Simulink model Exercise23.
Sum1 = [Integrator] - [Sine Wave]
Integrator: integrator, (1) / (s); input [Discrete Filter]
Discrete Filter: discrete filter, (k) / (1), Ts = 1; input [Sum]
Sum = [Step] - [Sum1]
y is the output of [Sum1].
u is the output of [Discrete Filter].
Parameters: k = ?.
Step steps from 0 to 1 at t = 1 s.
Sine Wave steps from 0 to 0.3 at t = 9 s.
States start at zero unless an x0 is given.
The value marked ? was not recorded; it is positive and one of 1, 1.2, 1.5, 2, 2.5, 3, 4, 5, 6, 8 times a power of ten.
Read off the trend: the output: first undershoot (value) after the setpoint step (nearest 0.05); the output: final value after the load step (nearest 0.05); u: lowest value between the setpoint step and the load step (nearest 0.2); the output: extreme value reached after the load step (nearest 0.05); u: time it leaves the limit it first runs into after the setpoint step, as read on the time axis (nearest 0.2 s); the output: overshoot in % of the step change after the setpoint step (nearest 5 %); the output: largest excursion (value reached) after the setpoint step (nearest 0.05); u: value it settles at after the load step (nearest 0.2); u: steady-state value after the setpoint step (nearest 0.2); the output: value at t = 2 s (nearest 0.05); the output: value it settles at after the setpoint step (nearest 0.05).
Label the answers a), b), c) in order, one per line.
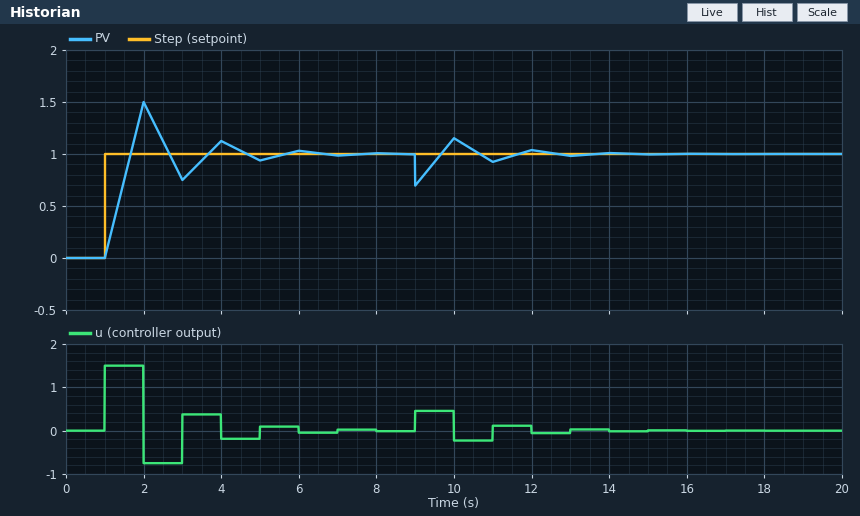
a) 0.75
b) 1.00
c) -0.8
d) 0.70
e) 2.0 s
f) 50 %
g) 1.50
h) 0.0
i) 0.0
j) 1.50
k) 1.00
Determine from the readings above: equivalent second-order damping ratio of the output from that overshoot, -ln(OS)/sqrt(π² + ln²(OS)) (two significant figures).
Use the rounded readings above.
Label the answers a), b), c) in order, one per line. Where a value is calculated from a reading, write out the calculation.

a) ln(0.5) = -0.693; 0.693 / sqrt(9.870 + 0.480) = 0.22
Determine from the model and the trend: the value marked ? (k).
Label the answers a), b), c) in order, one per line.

a) 1.5
